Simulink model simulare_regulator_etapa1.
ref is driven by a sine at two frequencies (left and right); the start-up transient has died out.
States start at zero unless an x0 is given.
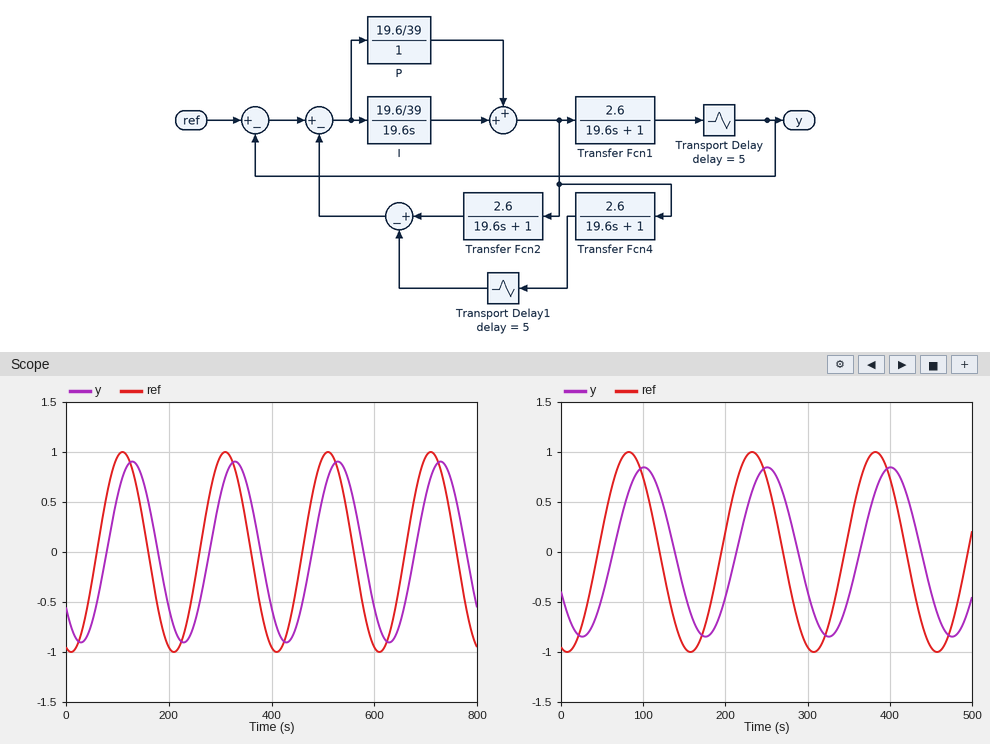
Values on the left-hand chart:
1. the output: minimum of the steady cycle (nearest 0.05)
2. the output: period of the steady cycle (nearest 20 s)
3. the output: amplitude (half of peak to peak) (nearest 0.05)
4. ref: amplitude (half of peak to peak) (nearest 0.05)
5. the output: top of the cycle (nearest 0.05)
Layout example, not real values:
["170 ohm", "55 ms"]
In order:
["-0.90", "200 s", "0.90", "1.00", "0.90"]
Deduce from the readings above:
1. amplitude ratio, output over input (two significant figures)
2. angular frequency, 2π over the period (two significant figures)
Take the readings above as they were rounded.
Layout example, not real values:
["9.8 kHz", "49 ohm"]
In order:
["0.90", "0.031 rad/s"]
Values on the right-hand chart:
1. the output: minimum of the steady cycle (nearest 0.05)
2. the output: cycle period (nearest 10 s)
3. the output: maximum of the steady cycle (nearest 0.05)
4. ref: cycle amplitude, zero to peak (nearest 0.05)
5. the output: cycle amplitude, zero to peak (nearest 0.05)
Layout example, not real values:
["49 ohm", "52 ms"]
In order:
["-0.85", "150 s", "0.85", "1.00", "0.85"]
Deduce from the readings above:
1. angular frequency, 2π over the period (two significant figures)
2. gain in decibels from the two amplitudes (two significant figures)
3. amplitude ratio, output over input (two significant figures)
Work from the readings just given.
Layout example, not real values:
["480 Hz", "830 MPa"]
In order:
["0.042 rad/s", "-1.4 dB", "0.85"]
